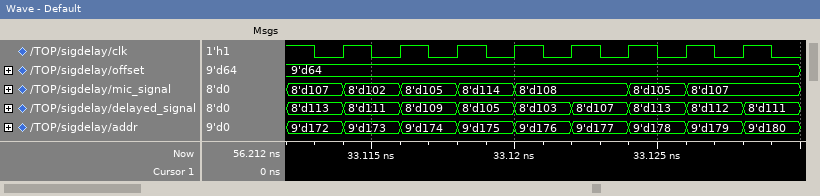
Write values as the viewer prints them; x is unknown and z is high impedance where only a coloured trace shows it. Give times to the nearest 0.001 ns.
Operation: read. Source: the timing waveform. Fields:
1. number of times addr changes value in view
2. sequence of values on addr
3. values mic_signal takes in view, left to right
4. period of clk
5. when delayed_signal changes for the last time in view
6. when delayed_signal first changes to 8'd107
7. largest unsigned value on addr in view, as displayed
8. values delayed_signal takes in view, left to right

8
9'd172, 9'd173, 9'd174, 9'd175, 9'd176, 9'd177, 9'd178, 9'd179, 9'd180
8'd107, 8'd102, 8'd105, 8'd114, 8'd108, 8'd105, 8'd107
0.002 ns
33.128 ns
33.122 ns
9'd180
8'd113, 8'd111, 8'd109, 8'd105, 8'd103, 8'd107, 8'd113, 8'd112, 8'd111
